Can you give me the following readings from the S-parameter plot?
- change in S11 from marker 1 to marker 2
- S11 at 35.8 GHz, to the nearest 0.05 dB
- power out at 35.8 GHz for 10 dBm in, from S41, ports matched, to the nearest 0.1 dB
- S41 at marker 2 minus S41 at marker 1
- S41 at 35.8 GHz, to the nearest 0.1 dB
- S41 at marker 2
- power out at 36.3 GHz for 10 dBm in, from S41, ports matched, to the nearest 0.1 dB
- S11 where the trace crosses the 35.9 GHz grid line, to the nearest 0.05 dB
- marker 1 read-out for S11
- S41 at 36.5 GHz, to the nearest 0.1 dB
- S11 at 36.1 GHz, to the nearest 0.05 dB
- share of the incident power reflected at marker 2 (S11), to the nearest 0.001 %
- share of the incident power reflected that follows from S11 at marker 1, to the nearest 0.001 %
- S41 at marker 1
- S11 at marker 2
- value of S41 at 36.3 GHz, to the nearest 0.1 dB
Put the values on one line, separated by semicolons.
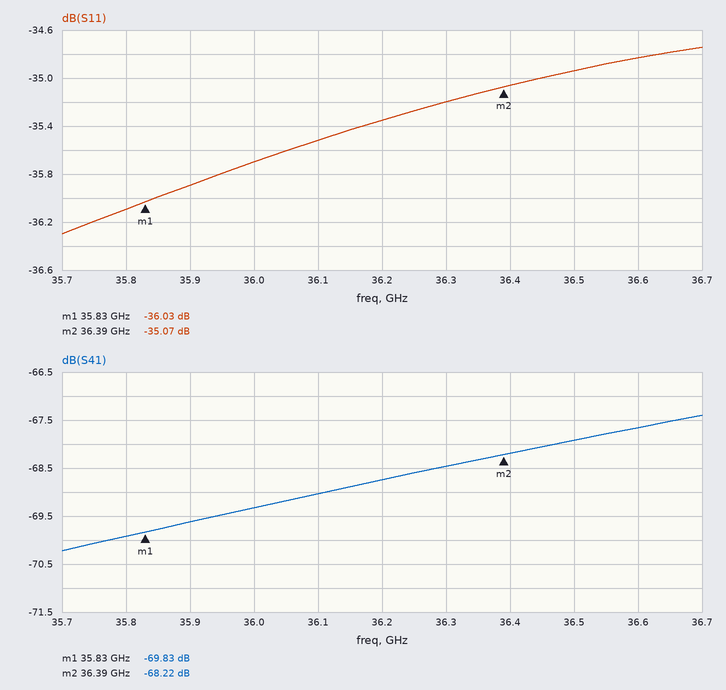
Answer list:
0.96 dB; -36.10 dB; -59.9 dBm; 1.61 dB; -69.9 dB; -68.22 dB; -58.5 dBm; -35.90 dB; -36.03 dB; -67.9 dB; -35.50 dB; 0.031 %; 0.025 %; -69.83 dB; -35.07 dB; -68.5 dB
